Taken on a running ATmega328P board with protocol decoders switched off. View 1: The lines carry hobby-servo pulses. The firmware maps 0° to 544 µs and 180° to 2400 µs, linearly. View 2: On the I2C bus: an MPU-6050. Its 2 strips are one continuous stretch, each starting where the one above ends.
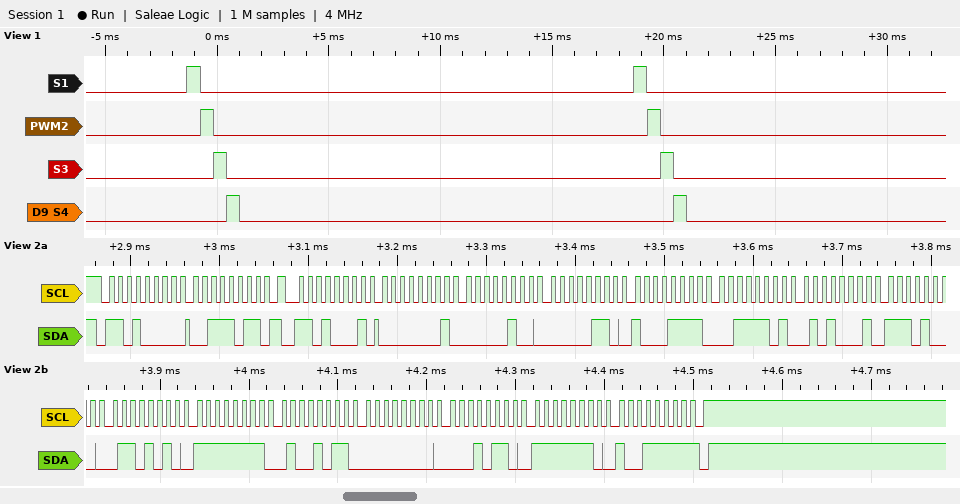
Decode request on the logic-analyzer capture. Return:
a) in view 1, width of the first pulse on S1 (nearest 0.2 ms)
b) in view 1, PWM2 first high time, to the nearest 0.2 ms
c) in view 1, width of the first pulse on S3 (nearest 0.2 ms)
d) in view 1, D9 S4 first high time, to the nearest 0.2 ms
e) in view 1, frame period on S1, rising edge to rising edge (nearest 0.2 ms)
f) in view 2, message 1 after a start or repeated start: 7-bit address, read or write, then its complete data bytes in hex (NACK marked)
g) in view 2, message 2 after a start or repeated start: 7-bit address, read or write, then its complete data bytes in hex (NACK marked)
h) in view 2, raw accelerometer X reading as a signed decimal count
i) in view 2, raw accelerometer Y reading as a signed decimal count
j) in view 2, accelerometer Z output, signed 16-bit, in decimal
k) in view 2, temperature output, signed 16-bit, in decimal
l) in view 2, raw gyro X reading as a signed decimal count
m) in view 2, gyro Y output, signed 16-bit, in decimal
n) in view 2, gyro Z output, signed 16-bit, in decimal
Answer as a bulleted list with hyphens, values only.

- 0.6 ms
- 0.6 ms
- 0.6 ms
- 0.6 ms
- 20.0 ms
- 0x68 write: 3B
- 0x68 read: 01 04 06 8F 3D 51 E8 6A FF 4B 00 16 FE 9F NACK
- 260
- 1679
- 15697
- -6038
- -181
- 22
- -353
